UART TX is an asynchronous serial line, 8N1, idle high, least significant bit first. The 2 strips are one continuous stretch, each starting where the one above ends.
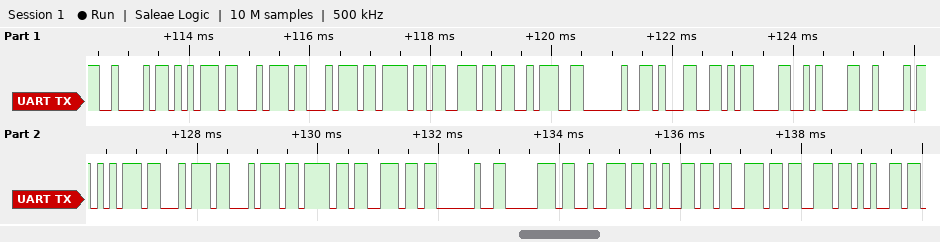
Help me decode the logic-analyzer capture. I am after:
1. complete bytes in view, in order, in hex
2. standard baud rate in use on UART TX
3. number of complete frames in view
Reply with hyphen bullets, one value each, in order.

- 42 75 74 74 6F 6E 3A 20 31 0D 0A 42 75 74 74 6F 6E 20 70 72 65 73 73 65
- 9600 baud
- 24
